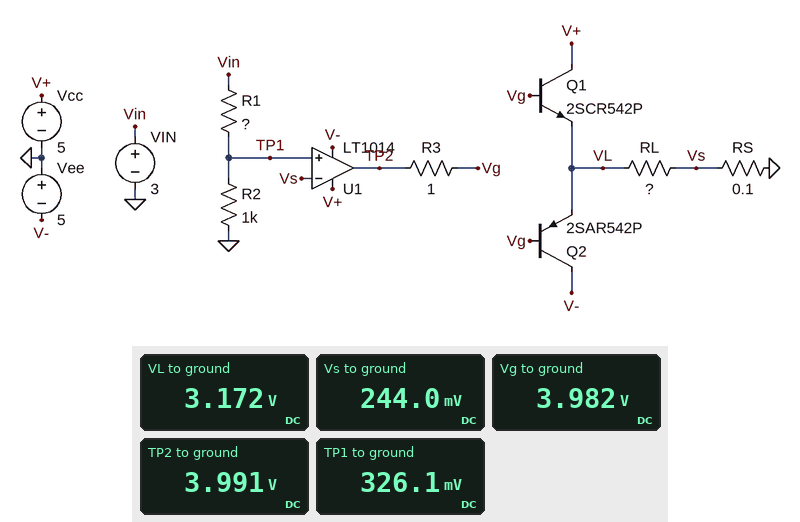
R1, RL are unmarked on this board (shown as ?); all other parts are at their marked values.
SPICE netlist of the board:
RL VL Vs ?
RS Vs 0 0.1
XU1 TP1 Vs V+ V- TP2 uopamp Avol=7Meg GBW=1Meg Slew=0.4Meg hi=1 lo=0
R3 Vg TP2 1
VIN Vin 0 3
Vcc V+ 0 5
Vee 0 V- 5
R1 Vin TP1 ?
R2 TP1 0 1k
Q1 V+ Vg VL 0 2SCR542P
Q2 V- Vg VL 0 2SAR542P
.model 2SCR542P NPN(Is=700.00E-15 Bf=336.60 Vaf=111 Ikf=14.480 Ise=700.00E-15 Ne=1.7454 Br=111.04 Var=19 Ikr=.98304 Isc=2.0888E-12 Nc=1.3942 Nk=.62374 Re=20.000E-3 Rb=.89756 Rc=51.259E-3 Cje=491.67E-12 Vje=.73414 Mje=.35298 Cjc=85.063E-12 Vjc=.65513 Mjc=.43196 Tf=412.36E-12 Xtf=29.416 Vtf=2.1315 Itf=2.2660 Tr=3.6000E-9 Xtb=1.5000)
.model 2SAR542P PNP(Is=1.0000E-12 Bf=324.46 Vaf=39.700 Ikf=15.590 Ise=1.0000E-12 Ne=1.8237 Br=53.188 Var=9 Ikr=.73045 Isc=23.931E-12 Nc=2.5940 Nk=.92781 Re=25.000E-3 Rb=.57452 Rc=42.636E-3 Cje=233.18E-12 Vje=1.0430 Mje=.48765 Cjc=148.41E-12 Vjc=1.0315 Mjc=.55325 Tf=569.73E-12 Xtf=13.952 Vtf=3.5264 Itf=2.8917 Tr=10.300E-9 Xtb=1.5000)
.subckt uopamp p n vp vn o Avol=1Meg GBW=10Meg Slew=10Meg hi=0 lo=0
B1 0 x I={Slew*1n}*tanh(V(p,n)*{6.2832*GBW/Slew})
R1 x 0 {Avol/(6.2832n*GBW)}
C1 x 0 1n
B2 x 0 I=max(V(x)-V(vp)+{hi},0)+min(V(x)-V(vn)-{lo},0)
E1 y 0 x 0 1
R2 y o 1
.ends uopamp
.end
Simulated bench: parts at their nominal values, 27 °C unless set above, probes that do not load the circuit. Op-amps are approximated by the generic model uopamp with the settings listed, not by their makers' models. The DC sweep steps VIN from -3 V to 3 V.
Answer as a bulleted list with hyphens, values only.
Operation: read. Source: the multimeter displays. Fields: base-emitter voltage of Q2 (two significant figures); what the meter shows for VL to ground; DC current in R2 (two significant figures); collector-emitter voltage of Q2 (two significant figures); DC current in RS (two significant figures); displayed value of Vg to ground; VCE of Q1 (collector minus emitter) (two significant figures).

- 810 mV
- 3.172 V
- 330 µA
- -8.2 V
- 2.4 A
- 3.982 V
- 1.8 V
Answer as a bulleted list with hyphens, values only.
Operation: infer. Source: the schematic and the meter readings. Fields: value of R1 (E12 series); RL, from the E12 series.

- 8.2 kΩ
- 1.2 Ω
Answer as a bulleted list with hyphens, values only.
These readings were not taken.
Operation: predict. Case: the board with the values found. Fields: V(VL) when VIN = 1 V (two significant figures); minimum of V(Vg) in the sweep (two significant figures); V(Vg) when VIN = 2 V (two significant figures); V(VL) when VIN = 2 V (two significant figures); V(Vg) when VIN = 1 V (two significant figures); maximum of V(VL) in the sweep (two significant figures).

- 1.4 V
- -5.0 V
- 3.6 V
- 2.8 V
- 2.2 V
- 3.2 V
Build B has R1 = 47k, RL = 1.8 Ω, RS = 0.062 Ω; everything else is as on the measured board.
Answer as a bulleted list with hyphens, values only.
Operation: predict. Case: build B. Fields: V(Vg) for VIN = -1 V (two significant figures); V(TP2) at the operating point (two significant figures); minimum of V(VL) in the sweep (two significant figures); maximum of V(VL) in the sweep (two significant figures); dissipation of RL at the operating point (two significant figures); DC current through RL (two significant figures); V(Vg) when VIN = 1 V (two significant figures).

- -1.3 V
- 2.6 V
- -1.9 V
- 1.9 V
- 1.8 W
- 1.0 A
- 1.3 V
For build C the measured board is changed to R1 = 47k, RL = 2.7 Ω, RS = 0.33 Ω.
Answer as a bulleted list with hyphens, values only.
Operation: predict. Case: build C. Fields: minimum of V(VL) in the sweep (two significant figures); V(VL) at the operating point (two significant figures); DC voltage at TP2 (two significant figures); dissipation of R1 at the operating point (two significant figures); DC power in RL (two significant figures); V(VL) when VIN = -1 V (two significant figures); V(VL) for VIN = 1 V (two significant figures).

- -570 mV
- 570 mV
- 1.3 V
- 180 µW
- 97 mW
- -190 mV
- 190 mV
